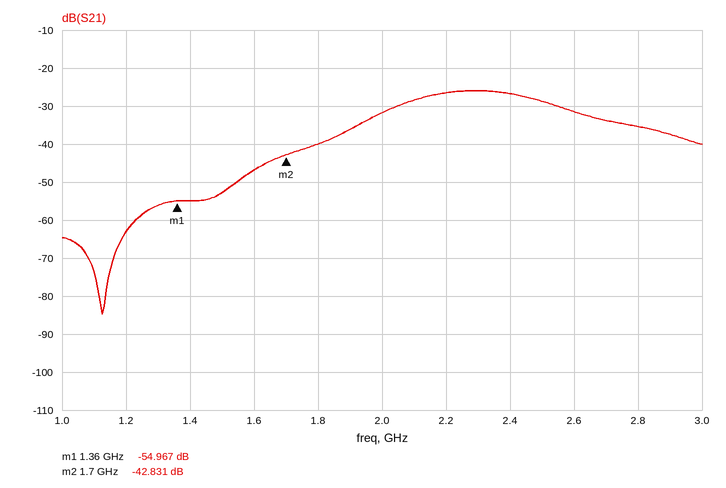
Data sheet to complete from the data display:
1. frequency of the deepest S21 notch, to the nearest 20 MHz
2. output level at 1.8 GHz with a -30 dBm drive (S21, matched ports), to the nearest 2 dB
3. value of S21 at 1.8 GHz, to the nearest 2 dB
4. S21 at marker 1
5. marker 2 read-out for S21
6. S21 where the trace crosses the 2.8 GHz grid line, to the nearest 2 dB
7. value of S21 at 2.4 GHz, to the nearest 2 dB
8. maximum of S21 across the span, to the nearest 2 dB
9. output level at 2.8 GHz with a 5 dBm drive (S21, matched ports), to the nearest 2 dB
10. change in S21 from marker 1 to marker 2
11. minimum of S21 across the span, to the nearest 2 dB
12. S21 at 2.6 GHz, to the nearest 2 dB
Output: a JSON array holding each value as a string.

["1.12 GHz", "-70 dBm", "-40 dB", "-54.967 dB", "-42.831 dB", "-36 dB", "-26 dB", "-26 dB", "-30 dBm", "12.136 dB", "-84 dB", "-32 dB"]
